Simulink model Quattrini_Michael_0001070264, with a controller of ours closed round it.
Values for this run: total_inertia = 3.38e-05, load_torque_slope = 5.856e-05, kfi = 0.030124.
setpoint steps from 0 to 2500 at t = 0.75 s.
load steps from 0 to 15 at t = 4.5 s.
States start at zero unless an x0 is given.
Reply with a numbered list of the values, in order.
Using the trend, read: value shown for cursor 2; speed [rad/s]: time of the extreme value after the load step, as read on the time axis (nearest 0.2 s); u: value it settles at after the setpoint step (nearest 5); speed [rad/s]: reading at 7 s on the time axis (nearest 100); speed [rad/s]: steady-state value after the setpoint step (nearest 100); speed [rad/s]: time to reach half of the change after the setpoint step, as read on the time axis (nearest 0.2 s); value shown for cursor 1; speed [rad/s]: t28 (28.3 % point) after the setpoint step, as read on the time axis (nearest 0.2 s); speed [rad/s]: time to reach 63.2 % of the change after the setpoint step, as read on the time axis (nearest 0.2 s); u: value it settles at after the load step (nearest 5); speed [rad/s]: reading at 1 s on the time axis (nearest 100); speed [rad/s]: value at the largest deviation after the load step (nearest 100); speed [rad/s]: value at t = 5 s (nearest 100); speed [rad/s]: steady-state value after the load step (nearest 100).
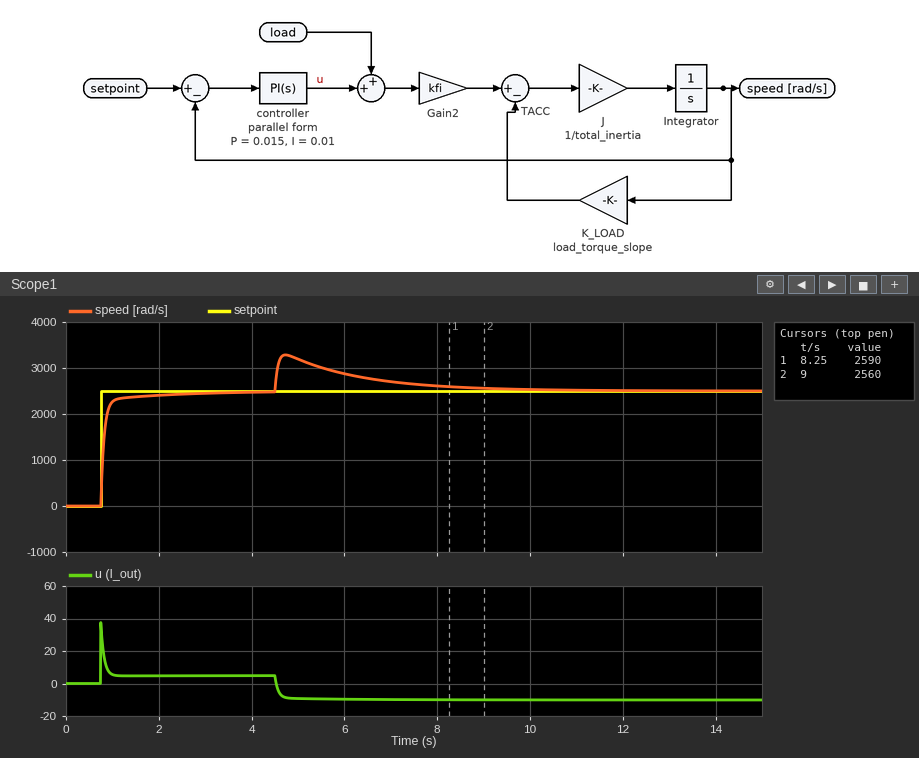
1. 2560
2. 4.8 s
3. 5
4. 2700
5. 2500
6. 0.8 s
7. 2590
8. 0.8 s
9. 0.8 s
10. -10
11. 2300
12. 3300
13. 3200
14. 2500
